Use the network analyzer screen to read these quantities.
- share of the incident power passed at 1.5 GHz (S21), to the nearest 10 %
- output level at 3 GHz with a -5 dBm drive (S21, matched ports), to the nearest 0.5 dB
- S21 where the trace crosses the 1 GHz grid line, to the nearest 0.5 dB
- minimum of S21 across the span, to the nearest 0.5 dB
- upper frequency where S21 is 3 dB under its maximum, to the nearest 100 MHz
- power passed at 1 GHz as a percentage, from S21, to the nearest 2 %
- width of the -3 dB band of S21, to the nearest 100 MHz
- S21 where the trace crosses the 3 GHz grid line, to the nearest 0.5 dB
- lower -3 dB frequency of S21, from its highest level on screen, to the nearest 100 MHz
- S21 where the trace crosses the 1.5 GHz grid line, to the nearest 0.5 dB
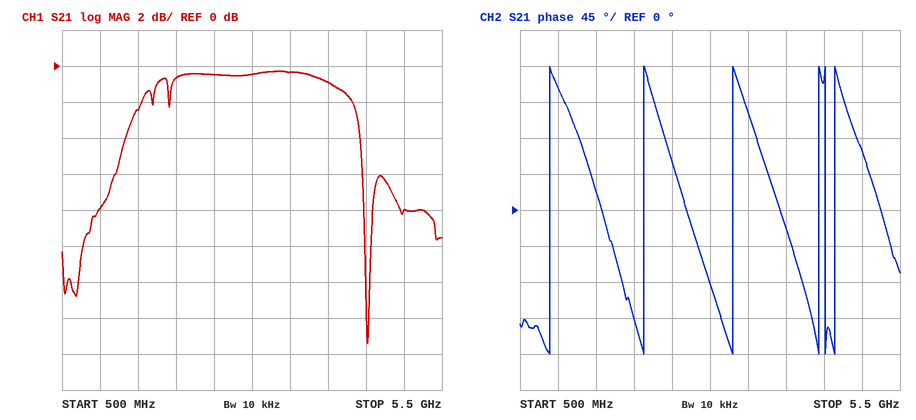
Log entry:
60 %
-5.5 dBm
-8.0 dB
-15.5 dB
4.4 GHz
16 %
3.0 GHz
-0.5 dB
1.4 GHz
-2.5 dB
